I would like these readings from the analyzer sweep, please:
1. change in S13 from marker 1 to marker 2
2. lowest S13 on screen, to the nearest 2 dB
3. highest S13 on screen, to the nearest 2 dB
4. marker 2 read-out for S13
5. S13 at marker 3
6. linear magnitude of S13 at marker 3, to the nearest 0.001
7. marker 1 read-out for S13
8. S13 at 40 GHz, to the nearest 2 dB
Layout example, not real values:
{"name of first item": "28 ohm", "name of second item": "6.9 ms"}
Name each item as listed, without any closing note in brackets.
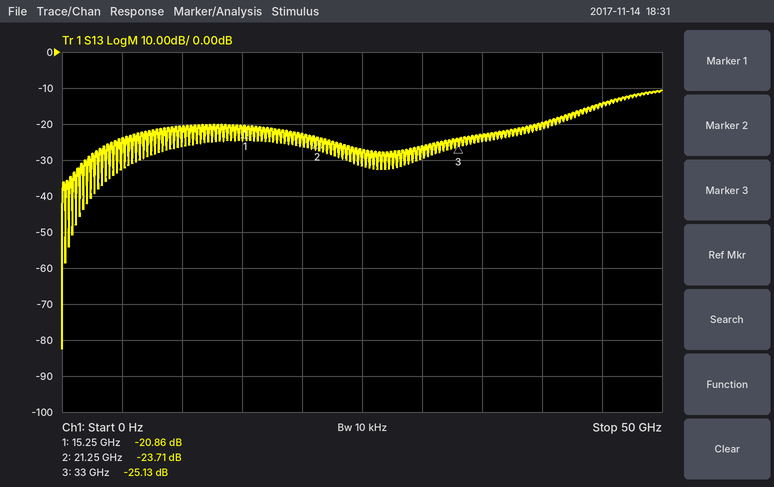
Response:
{"change in S13 from marker 1 to marker 2": "-2.85 dB", "lowest S13 on screen, to the nearest 2 dB": "-82 dB", "highest S13 on screen, to the nearest 2 dB": "-10 dB", "marker 2 read-out for S13": "-23.71 dB", "S13 at marker 3": "-25.13 dB", "linear magnitude of S13 at marker 3, to the nearest 0.001": "0.055", "marker 1 read-out for S13": "-20.86 dB", "S13 at 40 GHz, to the nearest 2 dB": "-20 dB"}
